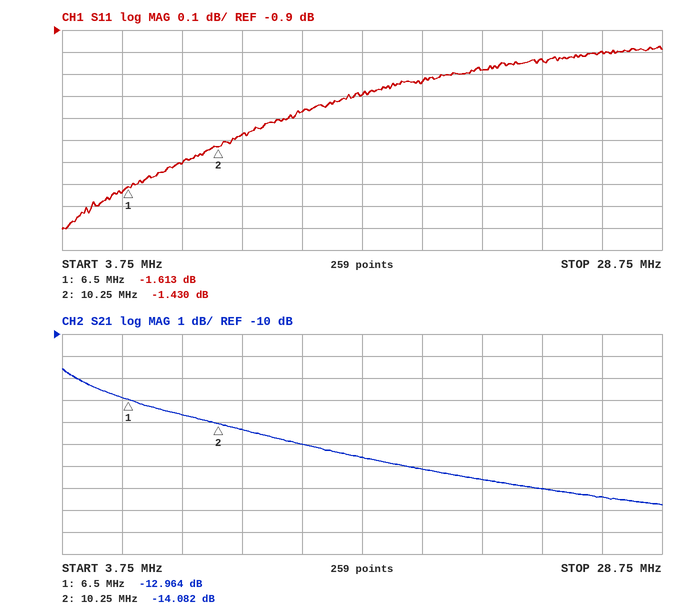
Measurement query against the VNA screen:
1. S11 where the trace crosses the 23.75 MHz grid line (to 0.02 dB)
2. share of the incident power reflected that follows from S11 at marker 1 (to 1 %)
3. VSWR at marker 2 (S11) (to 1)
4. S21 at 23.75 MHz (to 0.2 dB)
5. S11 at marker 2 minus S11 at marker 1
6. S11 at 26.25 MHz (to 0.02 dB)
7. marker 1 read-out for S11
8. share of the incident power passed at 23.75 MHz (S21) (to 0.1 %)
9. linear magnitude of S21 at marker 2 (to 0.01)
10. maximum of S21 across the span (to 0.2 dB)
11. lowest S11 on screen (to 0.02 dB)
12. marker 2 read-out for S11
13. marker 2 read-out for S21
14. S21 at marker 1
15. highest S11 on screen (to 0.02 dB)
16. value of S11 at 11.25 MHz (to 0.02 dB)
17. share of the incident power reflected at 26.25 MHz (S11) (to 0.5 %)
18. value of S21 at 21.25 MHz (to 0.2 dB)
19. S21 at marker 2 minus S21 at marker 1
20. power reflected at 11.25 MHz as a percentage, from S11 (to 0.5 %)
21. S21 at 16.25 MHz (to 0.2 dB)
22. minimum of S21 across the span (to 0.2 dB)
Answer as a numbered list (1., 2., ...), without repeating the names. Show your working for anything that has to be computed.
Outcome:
1. -1.04 dB
2. 10^(-1.613/10) ≈ 69 %
3. (1 + 0.8482)/(1 − 0.8482) ≈ 12
4. -17.0 dB
5. -1.43 − (-1.613) = 0.183 dB
6. -1.00 dB
7. -1.613 dB
8. 10^(-17/10) ≈ 2.0 %
9. 10^(-14.082/20) ≈ 0.20
10. -11.6 dB
11. -1.80 dB
12. -1.430 dB
13. -14.082 dB
14. -12.964 dB
15. -0.98 dB
16. -1.38 dB
17. 10^(-1/10) ≈ 79.4 %, so 79.5 % to the nearest 0.5 %
18. -16.6 dB
19. -14.082 − (-12.964) = -1.118 dB
20. 10^(-1.38/10) ≈ 72.8 %, so 73.0 % to the nearest 0.5 %
21. -15.6 dB
22. -17.8 dB
